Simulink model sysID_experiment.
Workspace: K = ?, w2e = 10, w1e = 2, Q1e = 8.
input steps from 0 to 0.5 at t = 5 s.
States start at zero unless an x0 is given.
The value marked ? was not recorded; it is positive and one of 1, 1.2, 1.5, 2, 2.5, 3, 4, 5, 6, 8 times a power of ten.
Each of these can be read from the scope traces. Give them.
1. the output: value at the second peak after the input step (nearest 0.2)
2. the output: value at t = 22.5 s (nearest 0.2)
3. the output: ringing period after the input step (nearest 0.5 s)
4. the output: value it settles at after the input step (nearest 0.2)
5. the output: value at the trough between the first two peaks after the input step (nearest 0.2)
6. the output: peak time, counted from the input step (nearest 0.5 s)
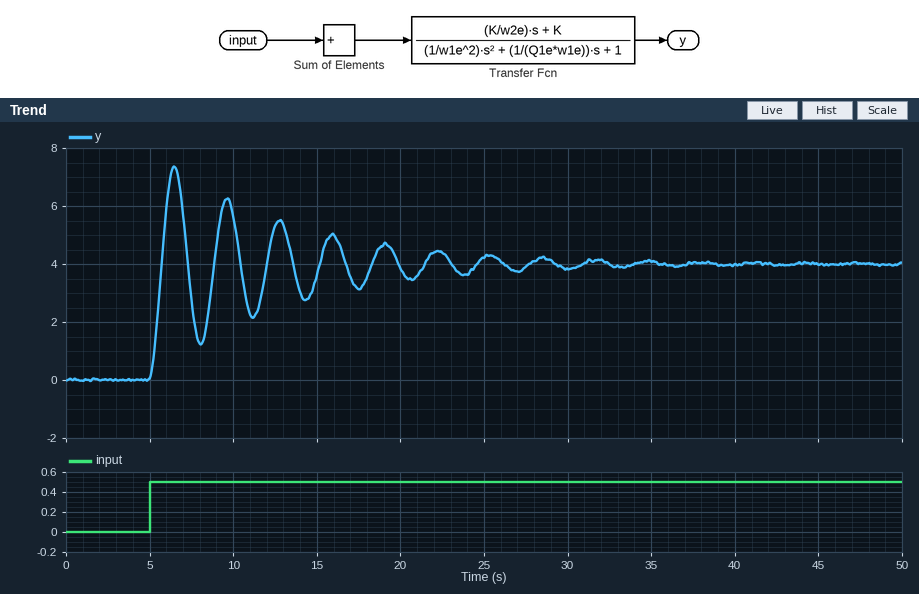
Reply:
6.2
4.4
3.0 s
4.0
1.2
1.5 s
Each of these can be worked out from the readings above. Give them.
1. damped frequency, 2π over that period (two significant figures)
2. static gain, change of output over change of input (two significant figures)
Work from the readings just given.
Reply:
2.1 rad/s
8.0
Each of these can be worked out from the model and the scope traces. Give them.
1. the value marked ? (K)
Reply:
8
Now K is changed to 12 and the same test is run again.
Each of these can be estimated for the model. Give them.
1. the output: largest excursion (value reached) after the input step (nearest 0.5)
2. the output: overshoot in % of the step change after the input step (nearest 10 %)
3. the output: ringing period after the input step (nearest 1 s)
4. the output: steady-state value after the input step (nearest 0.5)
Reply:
11.0
80 %
3 s
6.0
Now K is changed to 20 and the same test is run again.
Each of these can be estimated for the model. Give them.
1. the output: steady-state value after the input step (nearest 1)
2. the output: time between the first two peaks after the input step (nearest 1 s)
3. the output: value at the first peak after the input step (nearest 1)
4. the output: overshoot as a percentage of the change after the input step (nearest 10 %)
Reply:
10
3 s
18
80 %
